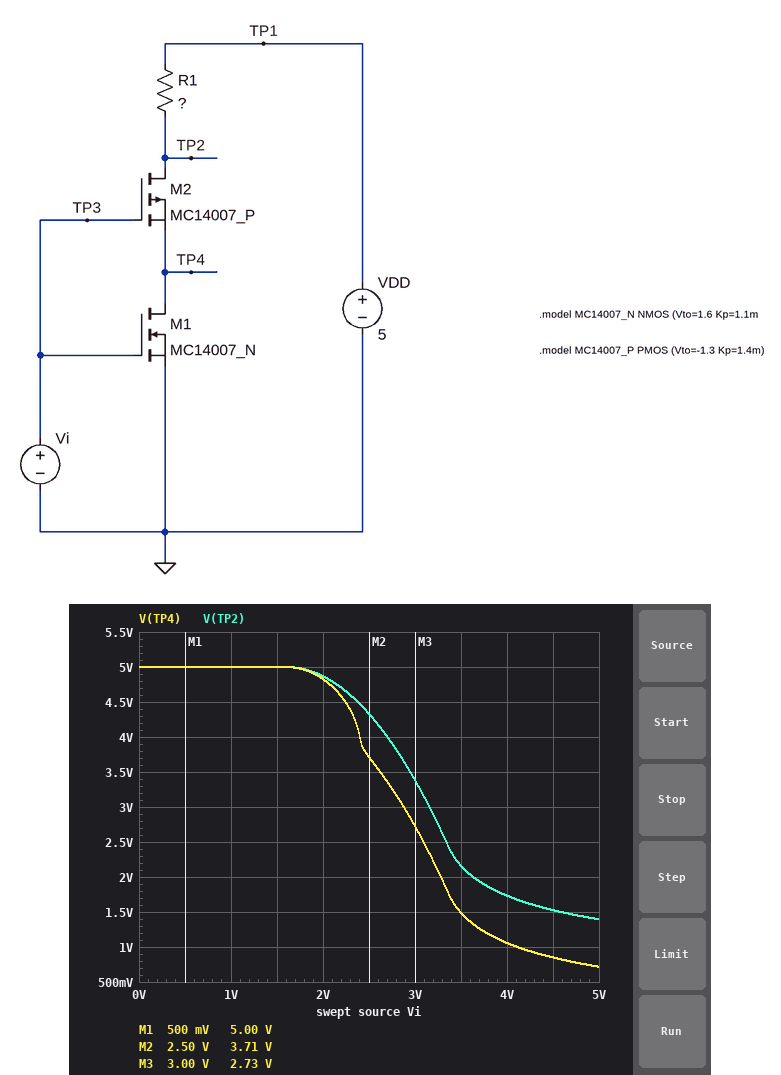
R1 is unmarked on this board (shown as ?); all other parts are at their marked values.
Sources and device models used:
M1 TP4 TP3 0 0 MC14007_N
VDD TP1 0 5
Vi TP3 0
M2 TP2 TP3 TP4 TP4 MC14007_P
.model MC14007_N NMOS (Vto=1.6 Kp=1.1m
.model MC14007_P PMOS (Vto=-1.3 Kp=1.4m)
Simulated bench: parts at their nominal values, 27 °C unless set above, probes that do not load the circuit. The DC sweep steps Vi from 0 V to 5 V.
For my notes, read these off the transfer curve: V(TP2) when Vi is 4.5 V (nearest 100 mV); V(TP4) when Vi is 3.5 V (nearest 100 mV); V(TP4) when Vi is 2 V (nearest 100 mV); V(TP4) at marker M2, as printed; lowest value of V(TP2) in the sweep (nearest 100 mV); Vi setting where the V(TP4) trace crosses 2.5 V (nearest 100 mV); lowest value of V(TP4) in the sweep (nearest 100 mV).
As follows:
1.5 V
1.5 V
4.8 V
3.71 V
1.4 V
3.1 V
700 mV
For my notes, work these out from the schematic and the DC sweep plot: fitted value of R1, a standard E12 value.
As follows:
1.5 kΩ
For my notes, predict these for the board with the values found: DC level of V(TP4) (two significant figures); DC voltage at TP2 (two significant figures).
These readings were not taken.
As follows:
5.0 V
5.0 V
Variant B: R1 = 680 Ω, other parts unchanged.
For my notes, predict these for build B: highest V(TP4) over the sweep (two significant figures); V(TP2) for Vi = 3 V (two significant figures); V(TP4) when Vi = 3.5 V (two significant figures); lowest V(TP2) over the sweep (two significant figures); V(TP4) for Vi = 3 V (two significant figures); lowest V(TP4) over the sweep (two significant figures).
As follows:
5.0 V
4.3 V
3.0 V
2.1 V
3.6 V
1.4 V
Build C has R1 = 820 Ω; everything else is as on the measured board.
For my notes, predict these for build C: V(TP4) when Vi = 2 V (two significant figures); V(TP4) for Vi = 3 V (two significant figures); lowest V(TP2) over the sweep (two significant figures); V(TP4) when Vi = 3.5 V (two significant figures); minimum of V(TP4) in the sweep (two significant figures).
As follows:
4.9 V
3.5 V
1.9 V
2.7 V
1.2 V
